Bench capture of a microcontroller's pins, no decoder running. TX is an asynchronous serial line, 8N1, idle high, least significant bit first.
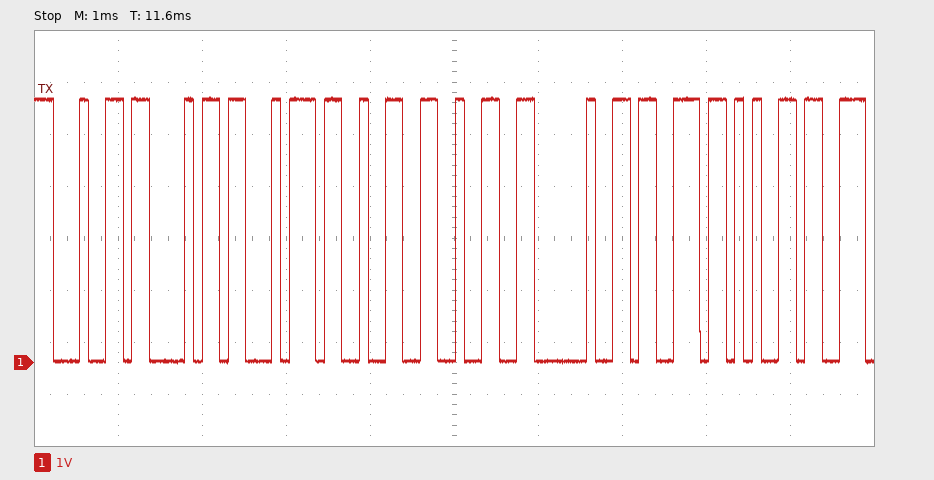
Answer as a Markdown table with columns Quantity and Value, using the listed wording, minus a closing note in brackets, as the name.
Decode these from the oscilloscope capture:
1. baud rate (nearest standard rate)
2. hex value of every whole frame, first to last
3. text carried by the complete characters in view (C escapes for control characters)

| Quantity | Value |
|---|---|
| baud rate | 9600 baud |
| hex value of every whole frame, first to last | 0x64 0x68 0x74 0x32 0x32 0x20 0x73 0x65 |
| text carried by the complete characters in view | "dht22 se" |
